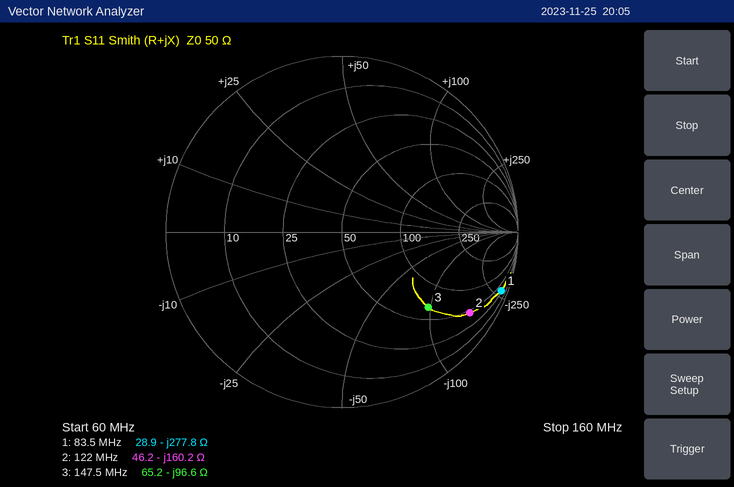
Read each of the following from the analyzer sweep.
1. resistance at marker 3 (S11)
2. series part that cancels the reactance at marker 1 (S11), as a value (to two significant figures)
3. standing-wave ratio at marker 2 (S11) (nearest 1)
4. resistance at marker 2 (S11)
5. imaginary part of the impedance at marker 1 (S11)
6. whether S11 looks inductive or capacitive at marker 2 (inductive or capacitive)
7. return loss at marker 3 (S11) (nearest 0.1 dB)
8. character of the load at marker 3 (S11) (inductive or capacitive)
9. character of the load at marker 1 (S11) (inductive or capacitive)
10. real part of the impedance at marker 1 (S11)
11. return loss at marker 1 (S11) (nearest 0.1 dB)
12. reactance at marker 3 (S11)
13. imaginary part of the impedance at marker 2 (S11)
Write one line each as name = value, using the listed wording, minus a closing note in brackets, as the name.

resistance at marker 3 = 65.2 Ω
series part that cancels the reactance at marker 1 (S11), as a value = 530 nH
standing-wave ratio at marker 2 (S11) = 13
resistance at marker 2 = 46.2 Ω
imaginary part of the impedance at marker 1 = -277.8 Ω
whether S11 looks inductive or capacitive at marker 2 = capacitive
return loss at marker 3 (S11) = 3.7 dB
character of the load at marker 3 (S11) = capacitive
character of the load at marker 1 (S11) = capacitive
real part of the impedance at marker 1 = 28.9 Ω
return loss at marker 1 (S11) = 0.3 dB
reactance at marker 3 = -96.6 Ω
imaginary part of the impedance at marker 2 = -160.2 Ω
